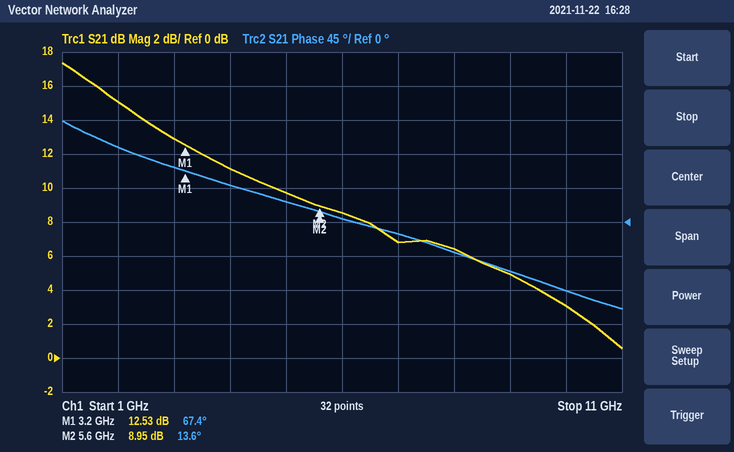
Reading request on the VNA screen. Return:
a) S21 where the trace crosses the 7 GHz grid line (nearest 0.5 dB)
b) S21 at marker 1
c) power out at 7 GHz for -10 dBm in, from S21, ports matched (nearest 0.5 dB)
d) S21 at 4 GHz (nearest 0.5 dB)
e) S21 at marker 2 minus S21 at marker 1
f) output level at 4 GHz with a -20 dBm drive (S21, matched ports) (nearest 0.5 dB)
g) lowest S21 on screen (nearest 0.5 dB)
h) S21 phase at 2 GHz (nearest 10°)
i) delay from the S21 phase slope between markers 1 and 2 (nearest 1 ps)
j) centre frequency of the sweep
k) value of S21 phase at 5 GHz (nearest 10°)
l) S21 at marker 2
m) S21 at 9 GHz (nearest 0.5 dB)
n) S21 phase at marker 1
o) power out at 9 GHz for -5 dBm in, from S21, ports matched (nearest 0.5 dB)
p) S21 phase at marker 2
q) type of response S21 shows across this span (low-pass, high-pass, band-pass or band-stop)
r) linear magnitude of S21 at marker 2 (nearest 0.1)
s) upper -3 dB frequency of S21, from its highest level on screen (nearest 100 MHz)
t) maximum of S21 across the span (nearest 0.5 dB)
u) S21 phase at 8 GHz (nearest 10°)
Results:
7.0 dB
12.53 dB
-3.0 dBm
11.0 dB
-3.58 dB
-9.0 dBm
0.5 dB
100°
62 ps
6 GHz
30°
8.95 dB
5.0 dB
67.4°
0.0 dBm
13.6°
low-pass
2.8
2.3 GHz
17.5 dB
-40°
